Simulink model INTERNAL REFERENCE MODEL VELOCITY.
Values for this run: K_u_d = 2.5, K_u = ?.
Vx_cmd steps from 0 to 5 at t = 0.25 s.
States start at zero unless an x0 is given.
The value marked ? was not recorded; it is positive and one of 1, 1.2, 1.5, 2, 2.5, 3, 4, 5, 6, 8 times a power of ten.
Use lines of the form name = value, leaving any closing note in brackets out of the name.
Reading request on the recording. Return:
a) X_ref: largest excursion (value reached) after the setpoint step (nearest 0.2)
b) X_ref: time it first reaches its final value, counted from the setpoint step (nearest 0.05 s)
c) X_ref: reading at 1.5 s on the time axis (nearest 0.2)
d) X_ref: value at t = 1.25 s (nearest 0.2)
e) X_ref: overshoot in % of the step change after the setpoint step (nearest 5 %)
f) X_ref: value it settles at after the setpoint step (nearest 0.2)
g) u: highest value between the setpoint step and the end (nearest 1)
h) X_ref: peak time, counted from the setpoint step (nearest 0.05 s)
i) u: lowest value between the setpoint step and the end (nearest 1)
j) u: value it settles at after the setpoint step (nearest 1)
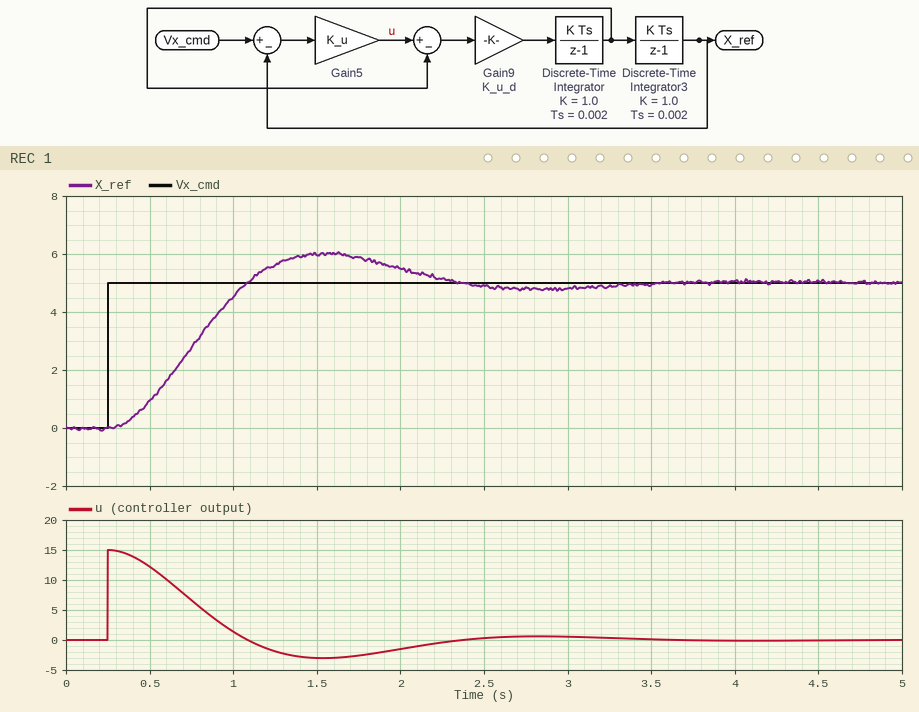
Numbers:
X_ref: largest excursion (value reached) after the setpoint step = 6.0
X_ref: time it first reaches its final value, counted from the setpoint step = 0.85 s
X_ref: reading at 1.5 s on the time axis = 6.0
X_ref: value at t = 1.25 s = 5.6
X_ref: overshoot in % of the step change after the setpoint step = 20 %
X_ref: value it settles at after the setpoint step = 5.0
u: highest value between the setpoint step and the end = 15
X_ref: peak time, counted from the setpoint step = 1.30 s
u: lowest value between the setpoint step and the end = -3
u: value it settles at after the setpoint step = 0
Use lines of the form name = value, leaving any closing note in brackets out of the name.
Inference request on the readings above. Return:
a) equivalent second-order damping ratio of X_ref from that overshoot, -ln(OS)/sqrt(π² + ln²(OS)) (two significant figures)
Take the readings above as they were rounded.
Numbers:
equivalent second-order damping ratio of X_ref from that overshoot, -ln(OS)/sqrt(π² + ln²(OS)) = 0.46
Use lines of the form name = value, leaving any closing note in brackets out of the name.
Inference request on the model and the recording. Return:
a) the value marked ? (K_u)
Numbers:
the value marked ? = 3
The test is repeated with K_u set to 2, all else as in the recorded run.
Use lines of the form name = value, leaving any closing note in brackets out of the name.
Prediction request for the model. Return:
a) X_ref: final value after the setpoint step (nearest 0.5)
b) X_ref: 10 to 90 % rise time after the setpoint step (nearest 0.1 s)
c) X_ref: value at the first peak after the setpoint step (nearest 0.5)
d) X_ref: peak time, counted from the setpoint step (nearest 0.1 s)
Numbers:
X_ref: final value after the setpoint step = 5.0
X_ref: 10 to 90 % rise time after the setpoint step = 0.8 s
X_ref: value at the first peak after the setpoint step = 5.5
X_ref: peak time, counted from the setpoint step = 1.7 s
